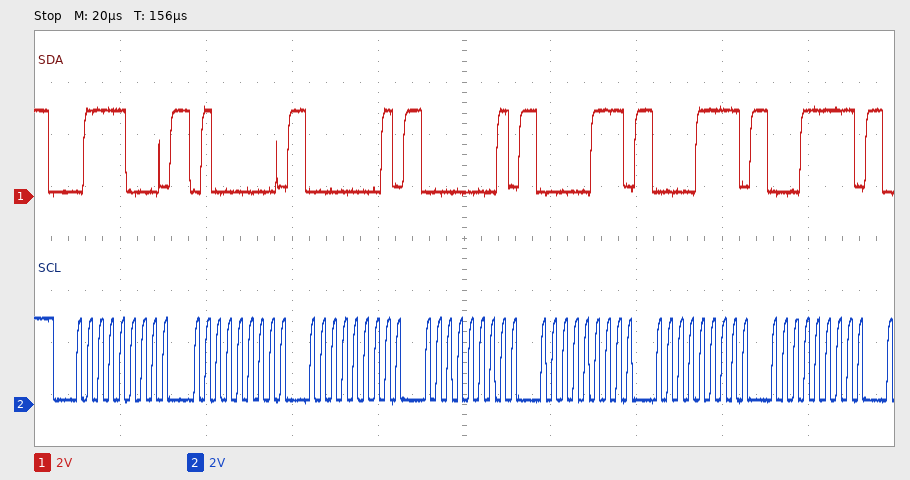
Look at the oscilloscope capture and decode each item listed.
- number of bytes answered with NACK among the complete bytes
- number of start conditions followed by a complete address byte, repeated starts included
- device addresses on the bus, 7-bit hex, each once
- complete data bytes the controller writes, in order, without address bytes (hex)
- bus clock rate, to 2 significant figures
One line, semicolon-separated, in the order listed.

0; 1; 0x3C; 40 01 01 07 0F 1F; 400 kHz
